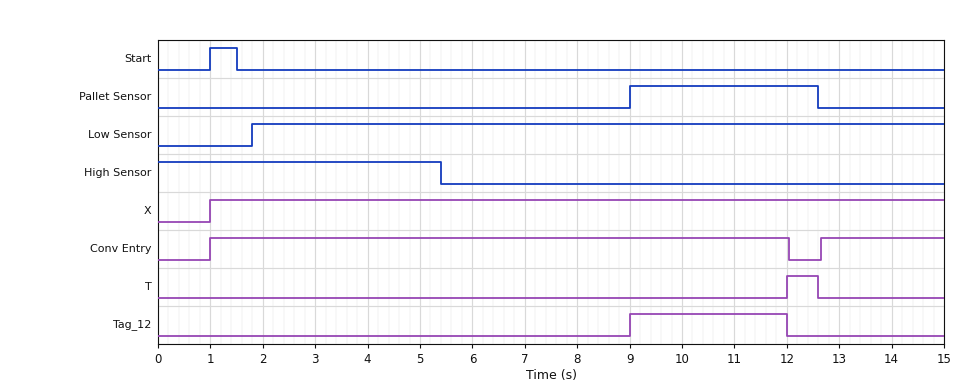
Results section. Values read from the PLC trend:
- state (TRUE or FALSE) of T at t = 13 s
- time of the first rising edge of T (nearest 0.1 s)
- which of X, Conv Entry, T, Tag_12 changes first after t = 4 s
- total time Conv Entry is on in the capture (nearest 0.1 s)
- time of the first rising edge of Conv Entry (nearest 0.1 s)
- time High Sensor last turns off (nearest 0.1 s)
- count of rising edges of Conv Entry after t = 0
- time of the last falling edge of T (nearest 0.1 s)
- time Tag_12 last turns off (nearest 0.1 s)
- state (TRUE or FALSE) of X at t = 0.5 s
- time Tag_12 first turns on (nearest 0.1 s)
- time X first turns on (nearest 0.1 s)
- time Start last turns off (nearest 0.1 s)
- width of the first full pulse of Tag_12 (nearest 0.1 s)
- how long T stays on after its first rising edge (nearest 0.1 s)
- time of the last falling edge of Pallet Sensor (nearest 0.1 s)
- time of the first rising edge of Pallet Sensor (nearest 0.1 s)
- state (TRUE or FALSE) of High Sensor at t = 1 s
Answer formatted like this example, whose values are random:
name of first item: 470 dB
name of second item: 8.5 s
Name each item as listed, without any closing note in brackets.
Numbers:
state (TRUE or FALSE) of T at t = 13 s: FALSE
time of the first rising edge of T: 12.0 s
which of X, Conv Entry, T, Tag_12 changes first after t = 4 s: Tag_12
total time Conv Entry is on in the capture: 13.4 s
time of the first rising edge of Conv Entry: 1.0 s
time High Sensor last turns off: 5.4 s
count of rising edges of Conv Entry after t = 0: 2
time of the last falling edge of T: 12.6 s
time Tag_12 last turns off: 12.0 s
state (TRUE or FALSE) of X at t = 0.5 s: FALSE
time Tag_12 first turns on: 9.0 s
time X first turns on: 1.0 s
time Start last turns off: 1.5 s
width of the first full pulse of Tag_12: 3.0 s
how long T stays on after its first rising edge: 0.6 s
time of the last falling edge of Pallet Sensor: 12.6 s
time of the first rising edge of Pallet Sensor: 9.0 s
state (TRUE or FALSE) of High Sensor at t = 1 s: TRUE
